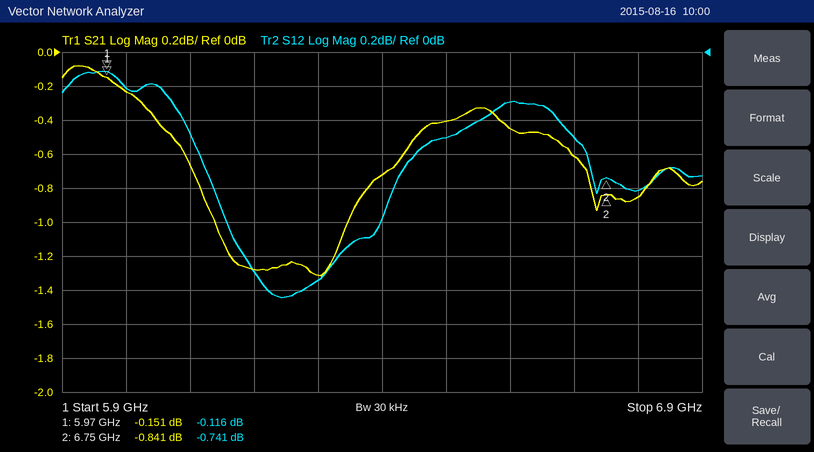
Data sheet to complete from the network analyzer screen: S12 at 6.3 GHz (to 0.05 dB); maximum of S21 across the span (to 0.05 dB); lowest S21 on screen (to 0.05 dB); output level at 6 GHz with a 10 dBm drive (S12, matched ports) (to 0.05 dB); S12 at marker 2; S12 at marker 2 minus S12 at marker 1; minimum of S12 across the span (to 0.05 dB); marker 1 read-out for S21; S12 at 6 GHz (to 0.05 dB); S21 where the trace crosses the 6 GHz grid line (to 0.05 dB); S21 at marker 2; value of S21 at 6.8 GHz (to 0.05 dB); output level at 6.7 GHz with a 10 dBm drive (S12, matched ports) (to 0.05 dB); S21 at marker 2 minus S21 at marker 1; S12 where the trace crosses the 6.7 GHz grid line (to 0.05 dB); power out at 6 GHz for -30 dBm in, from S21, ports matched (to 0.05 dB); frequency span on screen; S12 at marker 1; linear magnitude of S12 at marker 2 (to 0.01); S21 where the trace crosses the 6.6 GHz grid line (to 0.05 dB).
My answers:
-1.35 dB
-0.10 dB
-1.30 dB
9.80 dBm
-0.741 dB
-0.625 dB
-1.45 dB
-0.151 dB
-0.20 dB
-0.25 dB
-0.841 dB
-0.85 dB
9.50 dBm
-0.690 dB
-0.50 dB
-30.25 dBm
1 GHz
-0.116 dB
0.92
-0.45 dB
